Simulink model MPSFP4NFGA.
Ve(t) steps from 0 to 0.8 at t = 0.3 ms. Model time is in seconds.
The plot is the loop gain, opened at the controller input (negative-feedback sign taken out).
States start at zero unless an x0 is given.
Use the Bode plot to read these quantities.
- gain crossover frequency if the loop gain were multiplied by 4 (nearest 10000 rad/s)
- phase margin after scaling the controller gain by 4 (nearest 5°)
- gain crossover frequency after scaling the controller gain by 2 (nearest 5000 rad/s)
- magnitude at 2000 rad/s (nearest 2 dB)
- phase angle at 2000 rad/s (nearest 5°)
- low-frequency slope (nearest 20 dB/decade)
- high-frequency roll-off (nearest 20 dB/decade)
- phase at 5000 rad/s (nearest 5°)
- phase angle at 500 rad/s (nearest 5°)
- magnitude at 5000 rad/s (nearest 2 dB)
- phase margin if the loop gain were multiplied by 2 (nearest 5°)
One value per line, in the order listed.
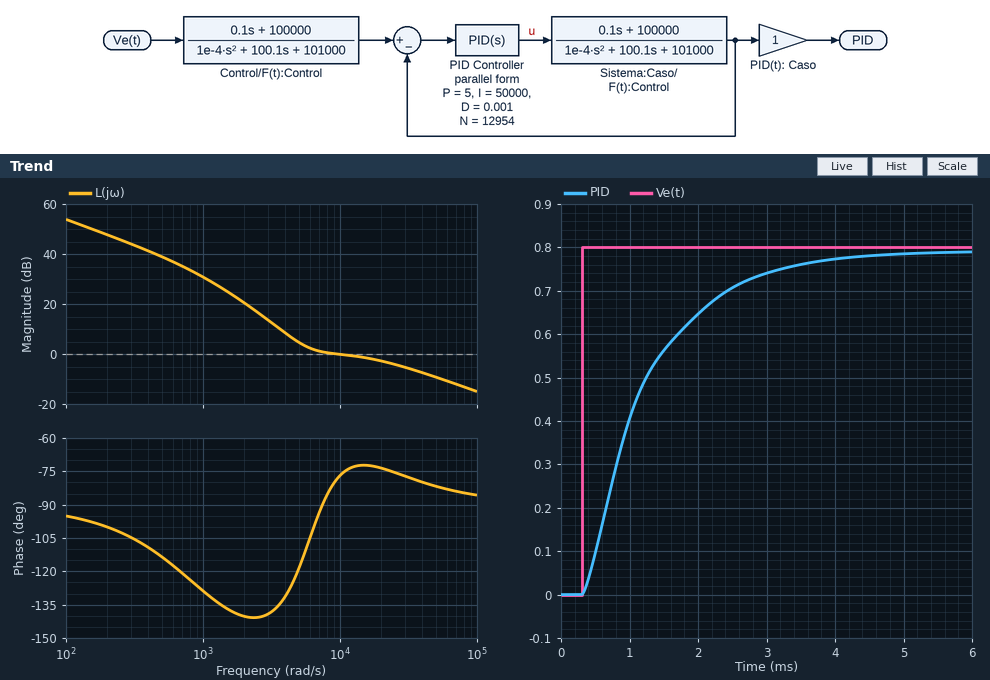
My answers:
70000 rad/s
95°
35000 rad/s
20 dB
-140°
-20 dB/decade
-20 dB/decade
-120°
-115°
4 dB
100°
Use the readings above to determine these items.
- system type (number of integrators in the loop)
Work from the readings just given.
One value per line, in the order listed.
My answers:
1
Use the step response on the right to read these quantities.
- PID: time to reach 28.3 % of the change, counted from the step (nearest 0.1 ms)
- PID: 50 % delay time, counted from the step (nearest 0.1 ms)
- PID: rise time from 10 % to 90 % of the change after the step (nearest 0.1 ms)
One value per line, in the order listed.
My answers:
0.4 ms
0.7 ms
2.1 ms
